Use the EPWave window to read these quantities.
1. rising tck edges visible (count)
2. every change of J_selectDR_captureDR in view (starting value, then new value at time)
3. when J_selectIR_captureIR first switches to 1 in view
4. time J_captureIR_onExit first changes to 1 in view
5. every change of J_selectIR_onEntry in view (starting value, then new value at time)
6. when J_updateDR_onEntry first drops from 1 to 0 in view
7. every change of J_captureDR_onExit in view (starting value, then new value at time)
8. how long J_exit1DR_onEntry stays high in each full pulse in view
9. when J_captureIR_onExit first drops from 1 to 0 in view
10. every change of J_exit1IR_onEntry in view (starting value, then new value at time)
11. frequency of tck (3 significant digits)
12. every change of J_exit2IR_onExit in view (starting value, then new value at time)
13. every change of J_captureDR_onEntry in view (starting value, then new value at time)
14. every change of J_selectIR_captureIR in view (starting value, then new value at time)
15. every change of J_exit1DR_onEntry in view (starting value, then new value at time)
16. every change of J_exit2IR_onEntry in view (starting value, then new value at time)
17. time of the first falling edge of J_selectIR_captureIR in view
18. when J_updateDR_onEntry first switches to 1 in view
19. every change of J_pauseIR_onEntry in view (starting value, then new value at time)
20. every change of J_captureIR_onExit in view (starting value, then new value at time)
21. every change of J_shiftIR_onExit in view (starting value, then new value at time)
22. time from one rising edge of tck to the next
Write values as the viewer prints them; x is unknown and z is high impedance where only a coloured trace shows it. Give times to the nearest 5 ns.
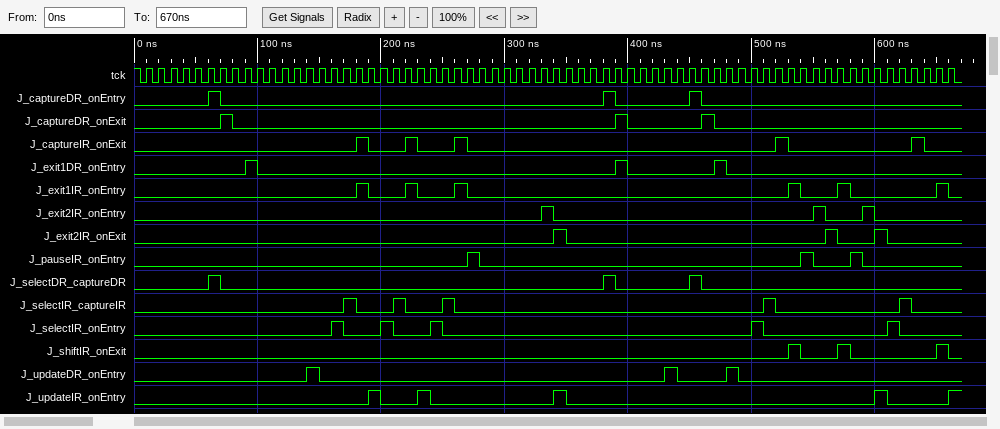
66
0, 1 at 60 ns, 0 at 70 ns, 1 at 380 ns, 0 at 390 ns, 1 at 450 ns, 0 at 460 ns
170 ns
180 ns
0, 1 at 160 ns, 0 at 170 ns, 1 at 200 ns, 0 at 210 ns, 1 at 240 ns, 0 at 250 ns, 1 at 500 ns, 0 at 510 ns, 1 at 610 ns, 0 at 620 ns
150 ns
0, 1 at 70 ns, 0 at 80 ns, 1 at 390 ns, 0 at 400 ns, 1 at 460 ns, 0 at 470 ns
10 ns, 10 ns, 10 ns
190 ns
0, 1 at 180 ns, 0 at 190 ns, 1 at 220 ns, 0 at 230 ns, 1 at 260 ns, 0 at 270 ns, 1 at 530 ns, 0 at 540 ns, 1 at 570 ns, 0 at 580 ns, 1 at 650 ns, 0 at 660 ns
100 MHz
0, 1 at 340 ns, 0 at 350 ns, 1 at 560 ns, 0 at 570 ns, 1 at 600 ns, 0 at 610 ns
0, 1 at 60 ns, 0 at 70 ns, 1 at 380 ns, 0 at 390 ns, 1 at 450 ns, 0 at 460 ns
0, 1 at 170 ns, 0 at 180 ns, 1 at 210 ns, 0 at 220 ns, 1 at 250 ns, 0 at 260 ns, 1 at 510 ns, 0 at 520 ns, 1 at 620 ns, 0 at 630 ns
0, 1 at 90 ns, 0 at 100 ns, 1 at 390 ns, 0 at 400 ns, 1 at 470 ns, 0 at 480 ns
0, 1 at 330 ns, 0 at 340 ns, 1 at 550 ns, 0 at 560 ns, 1 at 590 ns, 0 at 600 ns
180 ns
140 ns
0, 1 at 270 ns, 0 at 280 ns, 1 at 540 ns, 0 at 550 ns, 1 at 580 ns, 0 at 590 ns
0, 1 at 180 ns, 0 at 190 ns, 1 at 220 ns, 0 at 230 ns, 1 at 260 ns, 0 at 270 ns, 1 at 520 ns, 0 at 530 ns, 1 at 630 ns, 0 at 640 ns
0, 1 at 530 ns, 0 at 540 ns, 1 at 570 ns, 0 at 580 ns, 1 at 650 ns, 0 at 660 ns
10 ns
